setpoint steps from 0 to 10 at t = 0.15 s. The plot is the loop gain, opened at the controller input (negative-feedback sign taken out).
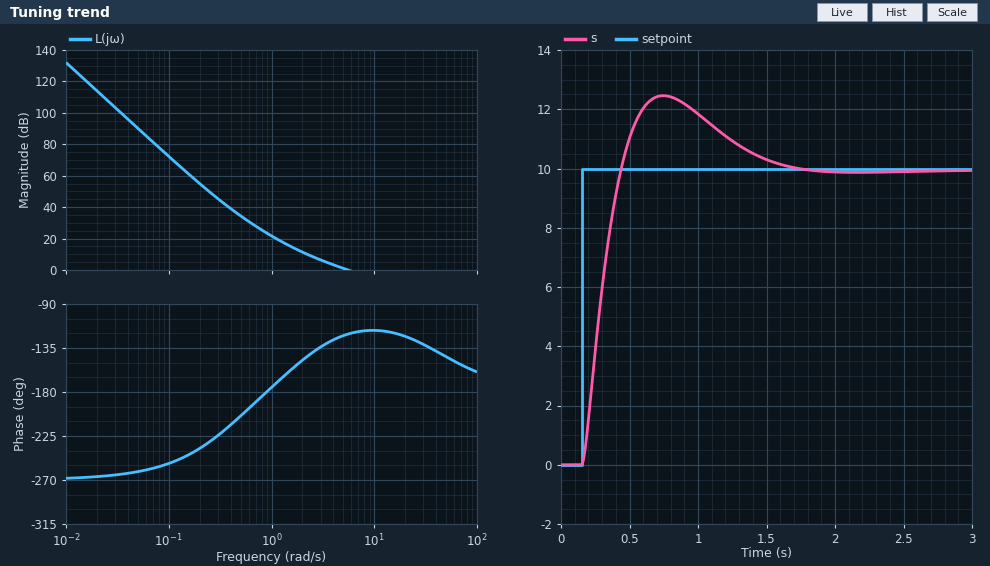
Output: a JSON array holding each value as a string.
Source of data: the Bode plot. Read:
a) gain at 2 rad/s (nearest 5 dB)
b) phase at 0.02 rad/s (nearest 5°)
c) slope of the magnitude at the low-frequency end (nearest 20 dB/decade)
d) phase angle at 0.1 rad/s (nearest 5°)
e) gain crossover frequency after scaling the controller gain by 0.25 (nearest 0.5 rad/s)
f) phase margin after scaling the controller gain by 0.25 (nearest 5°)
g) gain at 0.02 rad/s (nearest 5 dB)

["10 dB", "-265°", "-60 dB/decade", "-255°", "2.0 rad/s", "30°", "115 dB"]
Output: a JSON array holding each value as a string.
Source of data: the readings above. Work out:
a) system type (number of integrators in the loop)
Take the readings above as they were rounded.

["3"]
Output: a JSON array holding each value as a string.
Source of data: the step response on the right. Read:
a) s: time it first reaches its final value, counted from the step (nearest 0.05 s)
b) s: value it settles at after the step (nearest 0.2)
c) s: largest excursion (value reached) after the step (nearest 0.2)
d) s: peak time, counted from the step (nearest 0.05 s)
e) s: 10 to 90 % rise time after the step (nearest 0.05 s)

["0.30 s", "10.0", "12.4", "0.60 s", "0.20 s"]
